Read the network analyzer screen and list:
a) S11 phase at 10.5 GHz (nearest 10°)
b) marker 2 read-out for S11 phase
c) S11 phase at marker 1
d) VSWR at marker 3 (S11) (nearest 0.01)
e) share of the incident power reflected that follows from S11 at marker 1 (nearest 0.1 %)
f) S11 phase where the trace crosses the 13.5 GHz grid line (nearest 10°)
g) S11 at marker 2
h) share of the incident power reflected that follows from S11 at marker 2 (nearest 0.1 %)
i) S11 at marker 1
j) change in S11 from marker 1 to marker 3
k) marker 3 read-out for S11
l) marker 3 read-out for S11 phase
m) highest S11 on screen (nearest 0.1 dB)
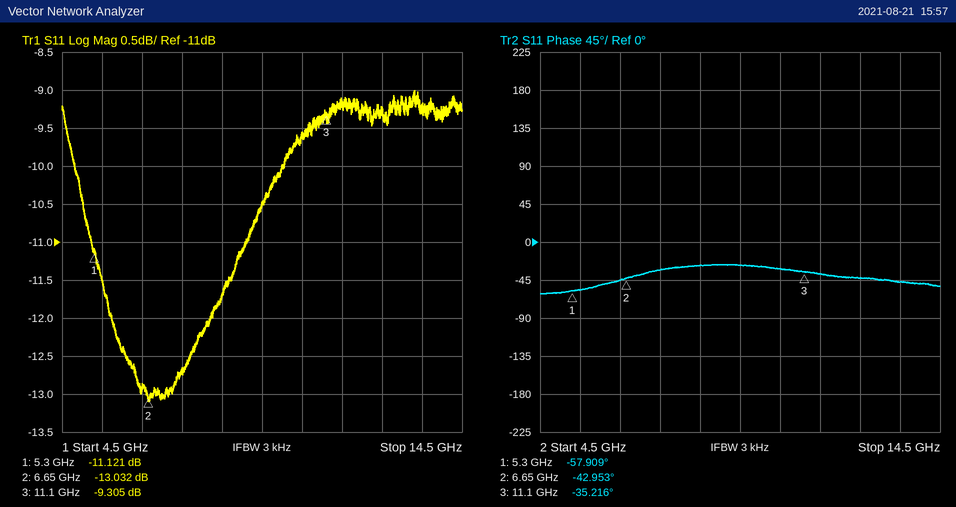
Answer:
-30°
-42.953°
-57.909°
2.04
7.7 %
-50°
-13.032 dB
5.0 %
-11.121 dB
1.816 dB
-9.305 dB
-35.216°
-9.0 dB
